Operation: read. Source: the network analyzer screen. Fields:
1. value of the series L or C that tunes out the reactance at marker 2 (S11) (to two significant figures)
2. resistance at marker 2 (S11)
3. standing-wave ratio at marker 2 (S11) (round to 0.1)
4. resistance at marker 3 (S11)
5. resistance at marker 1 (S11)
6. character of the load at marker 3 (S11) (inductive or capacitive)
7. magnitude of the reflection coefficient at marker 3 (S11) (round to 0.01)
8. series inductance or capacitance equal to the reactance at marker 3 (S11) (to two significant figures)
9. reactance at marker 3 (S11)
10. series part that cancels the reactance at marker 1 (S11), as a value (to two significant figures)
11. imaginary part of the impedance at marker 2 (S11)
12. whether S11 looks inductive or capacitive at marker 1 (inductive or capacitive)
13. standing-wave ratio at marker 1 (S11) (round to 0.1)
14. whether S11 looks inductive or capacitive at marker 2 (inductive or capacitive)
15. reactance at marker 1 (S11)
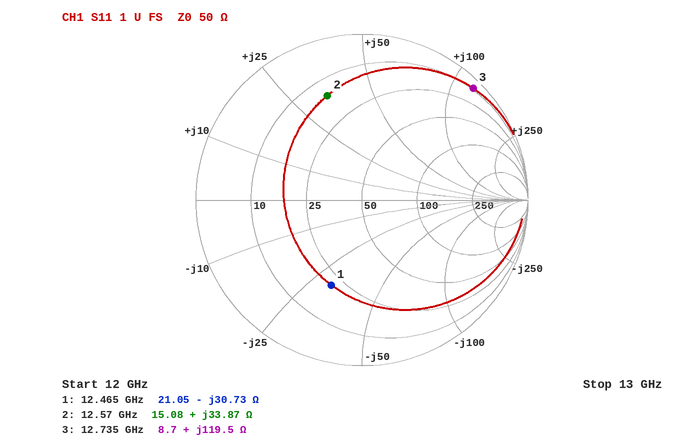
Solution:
370 fF
15.08 Ω
4.9
8.7 Ω
21.05 Ω
inductive
0.95
1.5 nH
+119.5 Ω
390 pH
+33.87 Ω
capacitive
3.4
inductive
-30.73 Ω
